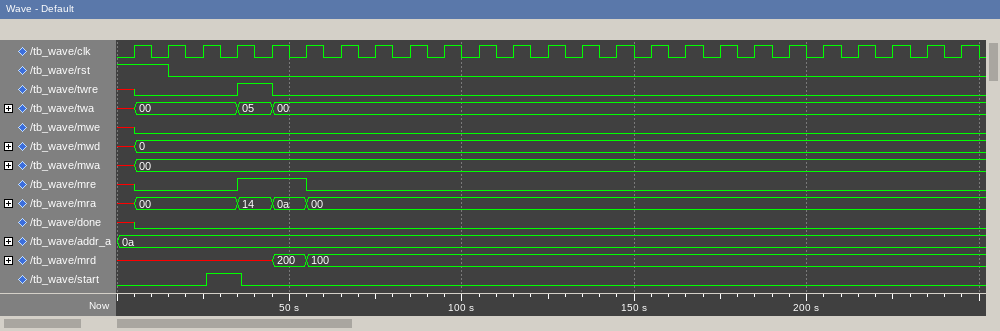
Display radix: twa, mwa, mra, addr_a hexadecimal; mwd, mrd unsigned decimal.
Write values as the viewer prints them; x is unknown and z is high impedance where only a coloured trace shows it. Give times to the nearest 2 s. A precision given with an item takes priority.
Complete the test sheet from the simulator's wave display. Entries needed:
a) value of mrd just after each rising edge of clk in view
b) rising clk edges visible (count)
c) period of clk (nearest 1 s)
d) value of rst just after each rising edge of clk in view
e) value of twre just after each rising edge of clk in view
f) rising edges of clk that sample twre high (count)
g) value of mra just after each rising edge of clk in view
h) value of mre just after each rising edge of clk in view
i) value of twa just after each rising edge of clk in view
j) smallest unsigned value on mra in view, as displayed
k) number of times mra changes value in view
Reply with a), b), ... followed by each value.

a) x, x, x, x, 200, 100, 100, 100, 100, 100, 100, 100, 100, 100, 100, 100, 100, 100, 100, 100, 100, 100, 100, 100, 100
b) 25
c) 10 s
d) 1 0 0 0 0 0 0 0 0 0 0 0 0 0 0 0 0 0 0 0 0 0 0 0 0
e) 0 0 0 1 0 0 0 0 0 0 0 0 0 0 0 0 0 0 0 0 0 0 0 0 0
f) 1
g) 00, 00, 00, 14, 0a, 00, 00, 00, 00, 00, 00, 00, 00, 00, 00, 00, 00, 00, 00, 00, 00, 00, 00, 00, 00
h) 0 0 0 1 1 0 0 0 0 0 0 0 0 0 0 0 0 0 0 0 0 0 0 0 0
i) 00, 00, 00, 05, 00, 00, 00, 00, 00, 00, 00, 00, 00, 00, 00, 00, 00, 00, 00, 00, 00, 00, 00, 00, 00
j) 00
k) 4
